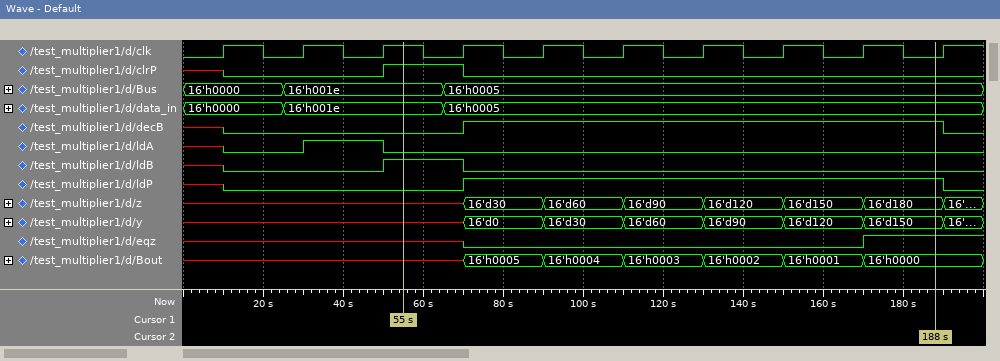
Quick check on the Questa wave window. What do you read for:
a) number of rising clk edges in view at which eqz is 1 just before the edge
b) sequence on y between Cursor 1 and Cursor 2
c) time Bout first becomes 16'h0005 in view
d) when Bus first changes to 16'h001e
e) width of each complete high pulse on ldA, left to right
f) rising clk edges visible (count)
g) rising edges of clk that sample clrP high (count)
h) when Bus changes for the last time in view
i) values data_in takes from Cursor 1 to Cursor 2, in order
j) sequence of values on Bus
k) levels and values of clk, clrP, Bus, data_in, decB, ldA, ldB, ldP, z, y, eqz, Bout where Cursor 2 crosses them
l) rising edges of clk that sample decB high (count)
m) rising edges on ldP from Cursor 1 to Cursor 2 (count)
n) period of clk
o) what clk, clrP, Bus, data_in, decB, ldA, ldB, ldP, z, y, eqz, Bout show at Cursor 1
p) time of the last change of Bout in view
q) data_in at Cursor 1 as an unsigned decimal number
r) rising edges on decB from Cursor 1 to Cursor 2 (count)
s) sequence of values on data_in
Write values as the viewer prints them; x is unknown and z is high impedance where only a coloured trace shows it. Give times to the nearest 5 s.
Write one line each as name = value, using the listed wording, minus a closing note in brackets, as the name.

number of rising clk edges in view at which eqz is 1 just before the edge = 1
sequence on y between Cursor 1 and Cursor 2 = x, 16'd0, 16'd30, 16'd60, 16'd90, 16'd120, 16'd150
time Bout first becomes 16'h0005 in view = 70 s
when Bus first changes to 16'h001e = 25 s
width of each complete high pulse on ldA, left to right = 20 s
rising clk edges visible = 10
rising edges of clk that sample clrP high = 1
when Bus changes for the last time in view = 65 s
values data_in takes from Cursor 1 to Cursor 2, in order = 16'h001e, 16'h0005
sequence of values on Bus = 16'h0000, 16'h001e, 16'h0005
levels and values of clk, clrP, Bus, data_in, decB, ldA, ldB, ldP, z, y, eqz, Bout where Cursor 2 crosses them = clk=0, clrP=0, Bus=16'h0005, data_in=16'h0005, decB=1, ldA=0, ldB=0, ldP=1, z=16'd180, y=16'd150, eqz=1, Bout=16'h0000
rising edges of clk that sample decB high = 6
rising edges on ldP from Cursor 1 to Cursor 2 = 1
period of clk = 20 s
what clk, clrP, Bus, data_in, decB, ldA, ldB, ldP, z, y, eqz, Bout show at Cursor 1 = clk=1, clrP=1, Bus=16'h001e, data_in=16'h001e, decB=0, ldA=0, ldB=1, ldP=0, z=x, y=x, eqz=x, Bout=x
time of the last change of Bout in view = 170 s
data_in at Cursor 1 as an unsigned decimal number = 30
rising edges on decB from Cursor 1 to Cursor 2 = 1
sequence of values on data_in = 16'h0000, 16'h001e, 16'h0005
